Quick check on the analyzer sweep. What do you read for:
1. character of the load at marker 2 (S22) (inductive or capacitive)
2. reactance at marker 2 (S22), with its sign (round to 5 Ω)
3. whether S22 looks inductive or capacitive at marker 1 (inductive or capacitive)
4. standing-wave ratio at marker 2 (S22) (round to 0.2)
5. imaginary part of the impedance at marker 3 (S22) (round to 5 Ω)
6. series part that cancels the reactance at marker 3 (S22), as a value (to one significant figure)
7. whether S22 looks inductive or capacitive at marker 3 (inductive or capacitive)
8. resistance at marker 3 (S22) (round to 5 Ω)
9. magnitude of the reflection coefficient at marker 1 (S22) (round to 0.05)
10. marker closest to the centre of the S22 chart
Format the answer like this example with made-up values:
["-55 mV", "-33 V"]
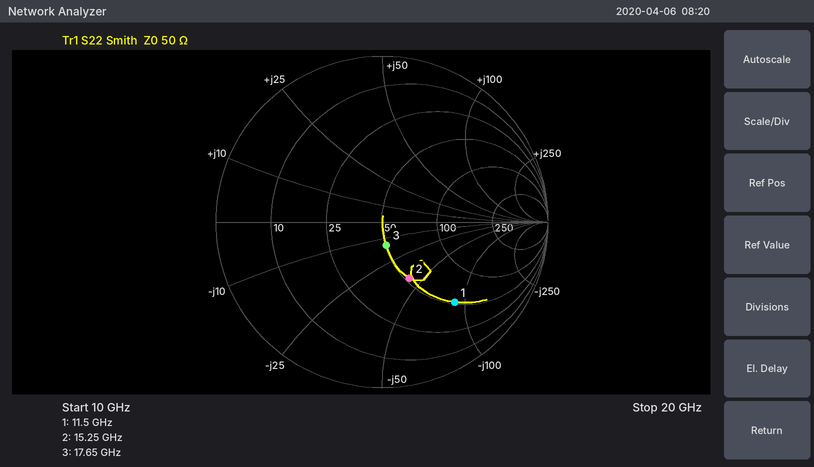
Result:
["capacitive", "-40 Ω", "capacitive", "2.2", "-15 Ω", "100 pH", "capacitive", "50 Ω", "0.65", "marker 3"]
